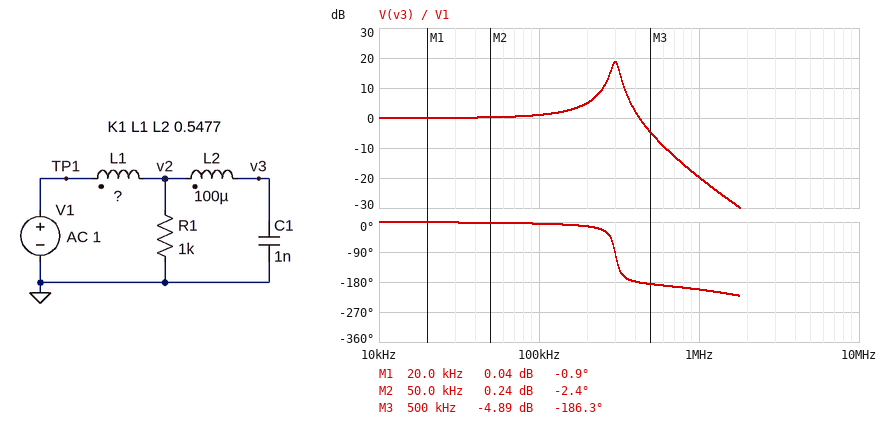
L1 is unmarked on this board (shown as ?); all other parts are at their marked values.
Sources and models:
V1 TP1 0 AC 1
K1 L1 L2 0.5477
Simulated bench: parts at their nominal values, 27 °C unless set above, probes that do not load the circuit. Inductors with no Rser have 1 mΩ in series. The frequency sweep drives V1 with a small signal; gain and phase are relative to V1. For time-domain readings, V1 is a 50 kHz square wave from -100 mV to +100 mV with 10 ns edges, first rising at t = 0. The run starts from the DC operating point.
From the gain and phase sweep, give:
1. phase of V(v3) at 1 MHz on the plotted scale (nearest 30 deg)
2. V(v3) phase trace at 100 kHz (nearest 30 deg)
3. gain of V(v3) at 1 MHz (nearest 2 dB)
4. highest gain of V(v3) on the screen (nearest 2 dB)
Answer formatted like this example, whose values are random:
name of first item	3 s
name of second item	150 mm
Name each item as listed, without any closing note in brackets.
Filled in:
phase of V(v3) at 1 MHz on the plotted scale	-210 deg
V(v3) phase trace at 100 kHz	0 deg
gain of V(v3) at 1 MHz	-20 dB
highest gain of V(v3) on the screen	18 dB
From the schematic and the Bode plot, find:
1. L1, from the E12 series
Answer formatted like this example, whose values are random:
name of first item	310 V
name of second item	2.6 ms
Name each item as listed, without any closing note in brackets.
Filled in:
L1, from the E12 series	82 µH
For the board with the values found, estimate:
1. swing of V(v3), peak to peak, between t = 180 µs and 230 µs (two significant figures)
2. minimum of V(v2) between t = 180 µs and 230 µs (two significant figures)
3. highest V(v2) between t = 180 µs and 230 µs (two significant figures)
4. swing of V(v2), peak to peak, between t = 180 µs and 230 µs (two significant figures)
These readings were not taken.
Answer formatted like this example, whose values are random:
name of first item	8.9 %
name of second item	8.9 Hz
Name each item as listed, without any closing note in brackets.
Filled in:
swing of V(v3), peak to peak, between t = 180 µs and 230 µs	450 mV
minimum of V(v2) between t = 180 µs and 230 µs	-160 mV
highest V(v2) between t = 180 µs and 230 µs	160 mV
swing of V(v2), peak to peak, between t = 180 µs and 230 µs	320 mV
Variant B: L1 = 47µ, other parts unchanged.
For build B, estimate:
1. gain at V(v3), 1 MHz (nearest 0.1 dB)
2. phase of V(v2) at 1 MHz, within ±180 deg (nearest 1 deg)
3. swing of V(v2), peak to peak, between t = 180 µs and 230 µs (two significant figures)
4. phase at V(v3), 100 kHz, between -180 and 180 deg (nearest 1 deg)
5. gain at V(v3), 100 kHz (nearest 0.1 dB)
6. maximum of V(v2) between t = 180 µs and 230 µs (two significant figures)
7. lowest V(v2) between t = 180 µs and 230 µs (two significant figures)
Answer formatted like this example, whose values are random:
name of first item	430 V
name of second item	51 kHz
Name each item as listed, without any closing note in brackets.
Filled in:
gain at V(v3), 1 MHz	-17.6 dB
phase of V(v2) at 1 MHz, within ±180 deg	-4 deg
swing of V(v2), peak to peak, between t = 180 µs and 230 µs	380 mV
phase at V(v3), 100 kHz, between -180 and 180 deg	-3 deg
gain at V(v3), 100 kHz	0.8 dB
maximum of V(v2) between t = 180 µs and 230 µs	190 mV
lowest V(v2) between t = 180 µs and 230 µs	-190 mV
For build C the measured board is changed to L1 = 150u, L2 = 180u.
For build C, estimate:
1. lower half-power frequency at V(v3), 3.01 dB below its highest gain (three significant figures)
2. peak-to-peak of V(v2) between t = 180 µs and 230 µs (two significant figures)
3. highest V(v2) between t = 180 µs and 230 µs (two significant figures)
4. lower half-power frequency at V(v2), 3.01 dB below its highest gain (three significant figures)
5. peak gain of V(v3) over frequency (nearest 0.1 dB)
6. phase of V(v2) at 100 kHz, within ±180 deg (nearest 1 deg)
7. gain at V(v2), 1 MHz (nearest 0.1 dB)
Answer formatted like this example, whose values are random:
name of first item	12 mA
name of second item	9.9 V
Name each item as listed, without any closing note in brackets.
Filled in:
lower half-power frequency at V(v3), 3.01 dB below its highest gain	204 kHz
peak-to-peak of V(v2) between t = 180 µs and 230 µs	330 mV
highest V(v2) between t = 180 µs and 230 µs	170 mV
lower half-power frequency at V(v2), 3.01 dB below its highest gain	195 kHz
peak gain of V(v3) over frequency	16.1 dB
phase of V(v2) at 100 kHz, within ±180 deg	-6 deg
gain at V(v2), 1 MHz	-6.1 dB
